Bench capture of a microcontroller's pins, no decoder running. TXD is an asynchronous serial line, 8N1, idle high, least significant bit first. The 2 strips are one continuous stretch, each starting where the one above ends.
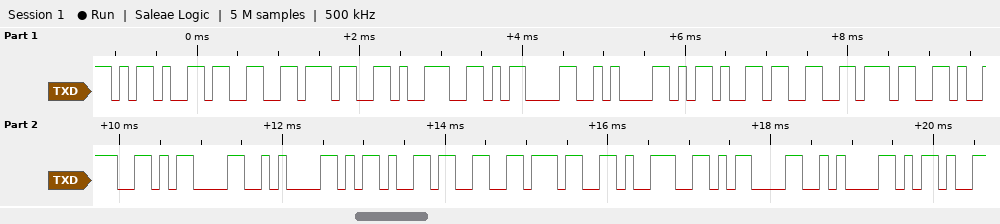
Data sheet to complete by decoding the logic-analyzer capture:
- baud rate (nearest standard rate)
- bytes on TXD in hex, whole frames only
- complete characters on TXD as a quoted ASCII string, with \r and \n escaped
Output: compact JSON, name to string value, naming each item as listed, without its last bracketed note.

{"baud rate": "9600 baud", "bytes on TXD in hex, whole frames only": "2D 33 37 39 0D 0A 2D 33 37 39 0D 0A 2D 33 37 39 0D 0A 2D", "complete characters on TXD as a quoted ASCII string, with \\r and \\n escaped": "\"-379\\r\\n-379\\r\\n-379\\r\\n-\""}
